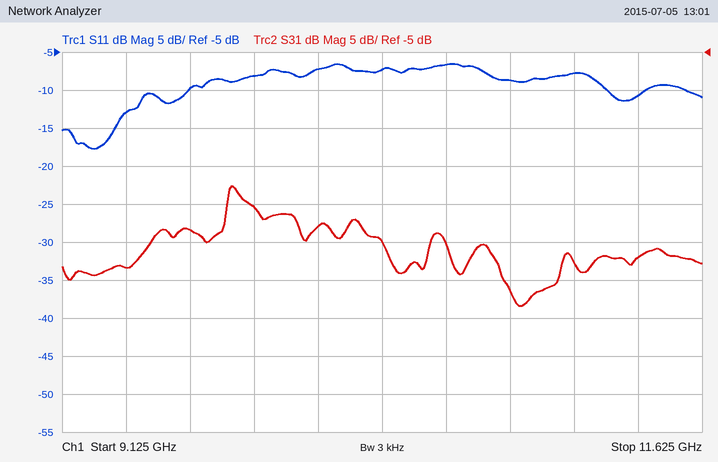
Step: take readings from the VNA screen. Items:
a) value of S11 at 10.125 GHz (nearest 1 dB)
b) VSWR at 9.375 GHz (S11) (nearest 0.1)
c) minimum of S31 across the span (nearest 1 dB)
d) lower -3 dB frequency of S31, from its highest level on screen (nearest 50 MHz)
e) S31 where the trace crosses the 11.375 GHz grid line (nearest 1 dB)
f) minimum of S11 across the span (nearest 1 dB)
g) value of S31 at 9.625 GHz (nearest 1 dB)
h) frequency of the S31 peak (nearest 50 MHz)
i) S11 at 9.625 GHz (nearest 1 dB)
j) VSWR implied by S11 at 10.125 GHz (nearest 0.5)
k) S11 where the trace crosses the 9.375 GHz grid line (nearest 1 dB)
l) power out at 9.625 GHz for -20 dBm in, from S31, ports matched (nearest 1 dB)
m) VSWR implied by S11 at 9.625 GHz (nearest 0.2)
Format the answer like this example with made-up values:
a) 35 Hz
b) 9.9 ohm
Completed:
a) -7 dB
b) 1.6
c) -38 dB
d) 9.75 GHz
e) -32 dB
f) -18 dB
g) -28 dB
h) 9.80 GHz
i) -10 dB
j) 2.5
k) -13 dB
l) -48 dBm
m) 2.0
